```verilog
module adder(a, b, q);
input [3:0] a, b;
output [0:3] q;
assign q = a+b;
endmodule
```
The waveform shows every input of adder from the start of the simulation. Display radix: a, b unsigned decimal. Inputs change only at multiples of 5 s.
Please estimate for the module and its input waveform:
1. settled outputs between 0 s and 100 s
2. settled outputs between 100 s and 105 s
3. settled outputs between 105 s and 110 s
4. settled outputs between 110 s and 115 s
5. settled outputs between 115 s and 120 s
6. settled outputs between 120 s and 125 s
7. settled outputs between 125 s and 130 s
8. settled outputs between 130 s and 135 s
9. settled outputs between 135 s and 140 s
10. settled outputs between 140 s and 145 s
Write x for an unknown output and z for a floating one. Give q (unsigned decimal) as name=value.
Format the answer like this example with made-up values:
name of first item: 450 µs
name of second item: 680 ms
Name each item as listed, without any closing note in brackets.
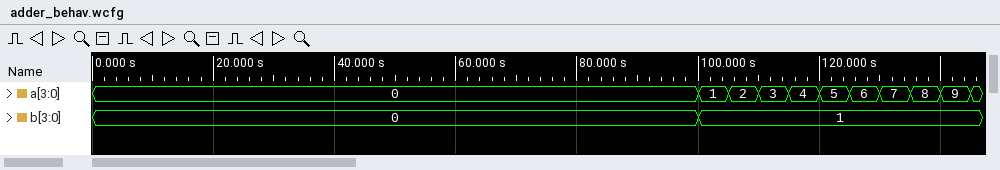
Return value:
settled outputs between 0 s and 100 s: q=0
settled outputs between 100 s and 105 s: q=2
settled outputs between 105 s and 110 s: q=3
settled outputs between 110 s and 115 s: q=4
settled outputs between 115 s and 120 s: q=5
settled outputs between 120 s and 125 s: q=6
settled outputs between 125 s and 130 s: q=7
settled outputs between 130 s and 135 s: q=8
settled outputs between 135 s and 140 s: q=9
settled outputs between 140 s and 145 s: q=10
